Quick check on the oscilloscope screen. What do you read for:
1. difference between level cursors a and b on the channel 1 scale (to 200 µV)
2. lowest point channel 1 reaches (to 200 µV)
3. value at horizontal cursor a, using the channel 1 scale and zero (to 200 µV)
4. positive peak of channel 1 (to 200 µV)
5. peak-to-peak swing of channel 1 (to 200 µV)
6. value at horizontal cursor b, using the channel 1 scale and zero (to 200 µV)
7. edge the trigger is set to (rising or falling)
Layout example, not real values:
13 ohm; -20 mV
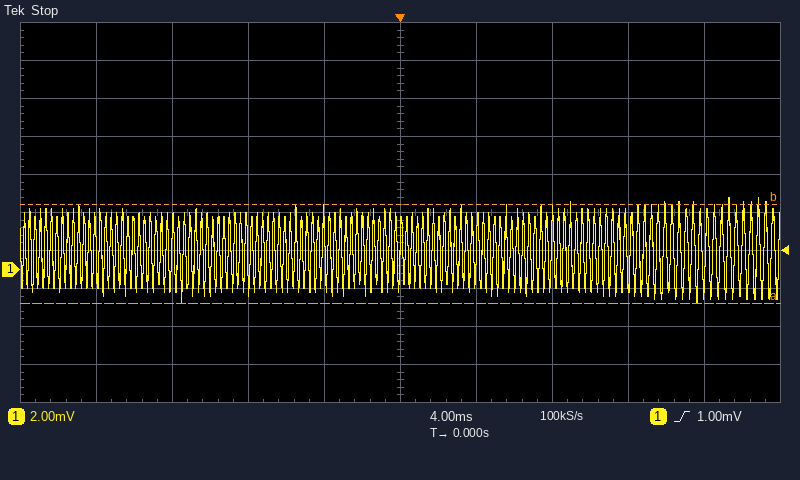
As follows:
5.2 mV; -1.8 mV; -1.8 mV; 3.8 mV; 5.6 mV; 3.4 mV; rising
